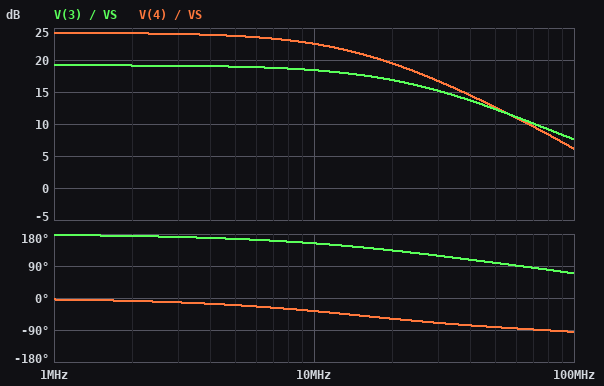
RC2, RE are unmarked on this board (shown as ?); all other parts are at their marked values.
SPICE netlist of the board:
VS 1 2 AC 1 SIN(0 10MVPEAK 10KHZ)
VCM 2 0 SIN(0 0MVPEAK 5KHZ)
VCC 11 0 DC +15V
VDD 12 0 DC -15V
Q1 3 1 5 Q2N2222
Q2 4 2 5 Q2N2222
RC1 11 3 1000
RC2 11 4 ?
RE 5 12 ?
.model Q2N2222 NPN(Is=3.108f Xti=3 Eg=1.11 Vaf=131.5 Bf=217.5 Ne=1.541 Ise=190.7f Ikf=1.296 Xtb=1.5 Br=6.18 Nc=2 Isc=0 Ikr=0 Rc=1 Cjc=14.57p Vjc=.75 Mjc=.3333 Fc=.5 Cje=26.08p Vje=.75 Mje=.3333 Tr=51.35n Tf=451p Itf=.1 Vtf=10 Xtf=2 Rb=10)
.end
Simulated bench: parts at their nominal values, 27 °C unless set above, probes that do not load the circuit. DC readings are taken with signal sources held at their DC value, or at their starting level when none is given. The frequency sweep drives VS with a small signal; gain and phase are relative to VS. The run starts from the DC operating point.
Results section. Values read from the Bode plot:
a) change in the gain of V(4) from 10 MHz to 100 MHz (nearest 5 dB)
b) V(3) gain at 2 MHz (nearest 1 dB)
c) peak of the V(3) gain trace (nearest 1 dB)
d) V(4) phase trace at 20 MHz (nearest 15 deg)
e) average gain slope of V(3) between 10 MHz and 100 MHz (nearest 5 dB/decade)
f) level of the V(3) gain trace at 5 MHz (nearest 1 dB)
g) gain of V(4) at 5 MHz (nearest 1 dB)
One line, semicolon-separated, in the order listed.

-15 dB; 19 dB; 19 dB; -60 deg; -10 dB/decade; 19 dB; 24 dB
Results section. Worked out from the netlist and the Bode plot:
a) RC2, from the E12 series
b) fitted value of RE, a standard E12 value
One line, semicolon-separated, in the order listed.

1.8 kΩ; 15 kΩ
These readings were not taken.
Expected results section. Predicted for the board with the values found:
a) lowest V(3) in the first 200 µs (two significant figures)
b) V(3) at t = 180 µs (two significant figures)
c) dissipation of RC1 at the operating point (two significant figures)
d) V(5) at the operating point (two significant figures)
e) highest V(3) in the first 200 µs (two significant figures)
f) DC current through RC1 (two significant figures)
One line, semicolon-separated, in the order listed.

14 V; 15 V; 220 µW; -660 mV; 15 V; 470 µA
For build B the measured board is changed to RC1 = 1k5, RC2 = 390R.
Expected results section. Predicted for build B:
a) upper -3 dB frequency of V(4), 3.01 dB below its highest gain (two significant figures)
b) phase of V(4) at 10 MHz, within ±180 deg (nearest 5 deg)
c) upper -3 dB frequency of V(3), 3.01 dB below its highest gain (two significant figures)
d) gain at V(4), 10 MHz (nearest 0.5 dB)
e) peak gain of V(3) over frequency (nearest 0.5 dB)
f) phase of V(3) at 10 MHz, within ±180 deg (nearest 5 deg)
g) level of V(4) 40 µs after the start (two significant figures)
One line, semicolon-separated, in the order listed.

53 MHz; -10 deg; 18 MHz; 10.5 dB; 22.5 dB; 145 deg; 15 V
